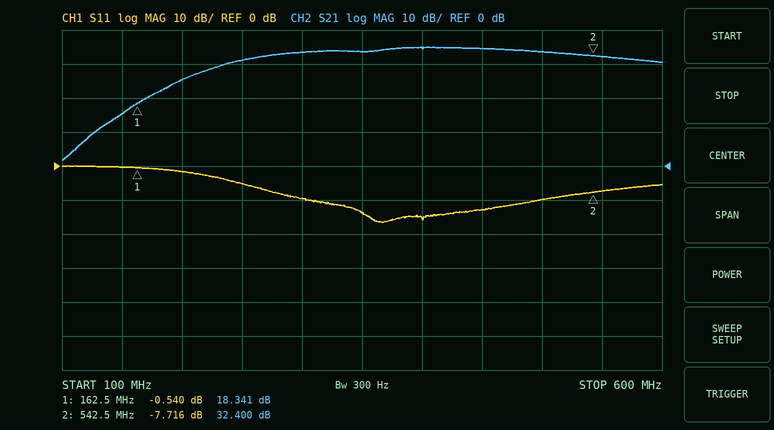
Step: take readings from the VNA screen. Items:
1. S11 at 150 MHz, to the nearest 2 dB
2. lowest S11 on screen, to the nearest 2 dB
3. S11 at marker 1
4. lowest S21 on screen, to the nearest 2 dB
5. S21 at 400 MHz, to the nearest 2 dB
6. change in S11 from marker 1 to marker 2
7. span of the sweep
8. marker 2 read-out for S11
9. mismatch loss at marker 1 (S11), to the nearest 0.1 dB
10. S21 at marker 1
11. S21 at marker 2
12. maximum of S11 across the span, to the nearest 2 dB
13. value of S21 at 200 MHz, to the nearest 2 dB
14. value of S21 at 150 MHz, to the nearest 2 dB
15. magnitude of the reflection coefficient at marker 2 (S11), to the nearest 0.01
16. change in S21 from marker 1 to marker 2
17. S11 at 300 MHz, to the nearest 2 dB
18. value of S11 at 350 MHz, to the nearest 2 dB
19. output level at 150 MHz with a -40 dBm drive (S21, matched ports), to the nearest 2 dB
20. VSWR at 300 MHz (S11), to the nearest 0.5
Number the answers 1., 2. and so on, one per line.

1. 0 dB
2. -16 dB
3. -0.540 dB
4. 2 dB
5. 34 dB
6. -7.176 dB
7. 500 MHz
8. -7.716 dB
9. 9.3 dB
10. 18.341 dB
11. 32.400 dB
12. 0 dB
13. 26 dB
14. 16 dB
15. 0.41
16. 14.059 dB
17. -10 dB
18. -14 dB
19. -24 dBm
20. 2.0
